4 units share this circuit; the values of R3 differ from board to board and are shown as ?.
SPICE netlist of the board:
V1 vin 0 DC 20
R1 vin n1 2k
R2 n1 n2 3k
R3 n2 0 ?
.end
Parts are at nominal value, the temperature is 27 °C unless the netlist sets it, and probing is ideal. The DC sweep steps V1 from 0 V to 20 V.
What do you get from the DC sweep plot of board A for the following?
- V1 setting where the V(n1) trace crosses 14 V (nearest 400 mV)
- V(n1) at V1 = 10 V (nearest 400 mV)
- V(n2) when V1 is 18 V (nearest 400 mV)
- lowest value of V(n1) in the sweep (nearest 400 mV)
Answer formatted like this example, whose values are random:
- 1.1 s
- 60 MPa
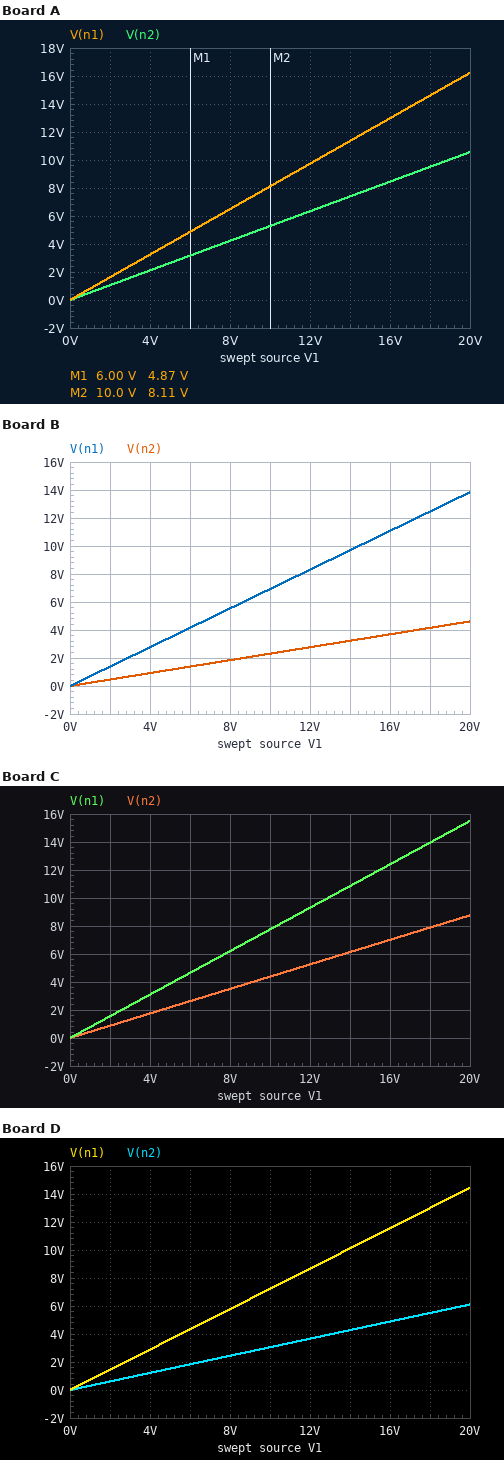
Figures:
- 17.2 V
- 8.0 V
- 9.6 V
- 0 V
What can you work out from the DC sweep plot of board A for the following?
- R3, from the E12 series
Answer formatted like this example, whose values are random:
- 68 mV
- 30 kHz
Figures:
- 5.6 kΩ
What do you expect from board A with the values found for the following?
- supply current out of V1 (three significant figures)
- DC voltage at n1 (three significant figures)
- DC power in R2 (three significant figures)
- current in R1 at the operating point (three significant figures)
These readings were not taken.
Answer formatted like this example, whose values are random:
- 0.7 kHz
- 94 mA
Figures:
- 1.89 mA
- 16.2 V
- 10.7 mW
- 1.89 mA
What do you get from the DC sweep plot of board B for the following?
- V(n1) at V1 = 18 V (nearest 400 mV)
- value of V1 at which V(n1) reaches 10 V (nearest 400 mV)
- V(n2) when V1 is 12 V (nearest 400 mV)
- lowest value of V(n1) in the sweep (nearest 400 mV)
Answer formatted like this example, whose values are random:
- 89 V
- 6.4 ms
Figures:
- 12.4 V
- 14.4 V
- 2.8 V
- 0 V
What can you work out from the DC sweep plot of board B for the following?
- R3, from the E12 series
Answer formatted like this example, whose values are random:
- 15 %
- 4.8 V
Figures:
- 1.5 kΩ
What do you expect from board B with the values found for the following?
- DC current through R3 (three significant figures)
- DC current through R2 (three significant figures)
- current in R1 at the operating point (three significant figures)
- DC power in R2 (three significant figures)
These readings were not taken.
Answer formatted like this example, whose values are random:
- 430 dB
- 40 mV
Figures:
- 3.08 mA
- 3.08 mA
- 3.08 mA
- 28.4 mW
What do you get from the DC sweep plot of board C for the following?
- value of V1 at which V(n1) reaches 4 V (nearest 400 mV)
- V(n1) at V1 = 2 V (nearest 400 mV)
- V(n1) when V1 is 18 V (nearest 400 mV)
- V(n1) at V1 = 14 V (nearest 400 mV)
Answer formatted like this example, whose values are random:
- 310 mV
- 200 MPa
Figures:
- 5.2 V
- 1.6 V
- 14.0 V
- 10.8 V
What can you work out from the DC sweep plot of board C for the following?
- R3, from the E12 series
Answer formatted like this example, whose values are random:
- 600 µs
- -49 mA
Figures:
- 3.9 kΩ
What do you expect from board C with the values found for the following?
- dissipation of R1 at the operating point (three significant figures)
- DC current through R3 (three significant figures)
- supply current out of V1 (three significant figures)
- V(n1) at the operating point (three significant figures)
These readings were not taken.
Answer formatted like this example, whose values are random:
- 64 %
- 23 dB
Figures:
- 10.1 mW
- 2.25 mA
- 2.25 mA
- 15.5 V
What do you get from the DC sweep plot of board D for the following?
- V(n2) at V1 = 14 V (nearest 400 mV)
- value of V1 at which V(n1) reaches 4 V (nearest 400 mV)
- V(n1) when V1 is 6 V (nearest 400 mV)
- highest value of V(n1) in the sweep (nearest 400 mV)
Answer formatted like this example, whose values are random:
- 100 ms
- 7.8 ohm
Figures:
- 4.4 V
- 5.6 V
- 4.4 V
- 14.4 V
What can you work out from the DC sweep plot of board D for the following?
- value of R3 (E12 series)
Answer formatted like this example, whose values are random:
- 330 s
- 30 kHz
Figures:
- 2.2 kΩ
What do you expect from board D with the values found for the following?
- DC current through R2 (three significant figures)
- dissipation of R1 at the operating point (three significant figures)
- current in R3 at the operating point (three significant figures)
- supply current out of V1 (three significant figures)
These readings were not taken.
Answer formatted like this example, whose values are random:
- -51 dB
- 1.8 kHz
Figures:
- 2.78 mA
- 15.4 mW
- 2.78 mA
- 2.78 mA
